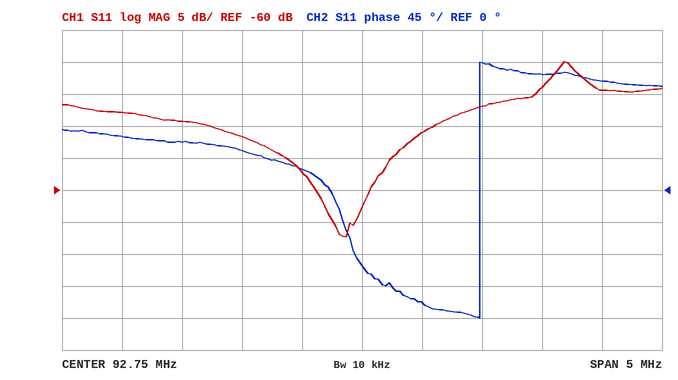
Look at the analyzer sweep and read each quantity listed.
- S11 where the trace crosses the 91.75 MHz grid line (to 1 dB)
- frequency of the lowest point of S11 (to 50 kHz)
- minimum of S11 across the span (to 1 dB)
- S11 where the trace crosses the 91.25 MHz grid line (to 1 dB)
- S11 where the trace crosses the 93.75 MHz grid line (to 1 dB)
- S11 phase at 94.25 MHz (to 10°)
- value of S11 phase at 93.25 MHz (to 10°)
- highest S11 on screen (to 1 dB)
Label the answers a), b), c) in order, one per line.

a) -52 dB
b) 92.60 MHz
c) -67 dB
d) -49 dB
e) -47 dB
f) 160°
g) -160°
h) -40 dB
